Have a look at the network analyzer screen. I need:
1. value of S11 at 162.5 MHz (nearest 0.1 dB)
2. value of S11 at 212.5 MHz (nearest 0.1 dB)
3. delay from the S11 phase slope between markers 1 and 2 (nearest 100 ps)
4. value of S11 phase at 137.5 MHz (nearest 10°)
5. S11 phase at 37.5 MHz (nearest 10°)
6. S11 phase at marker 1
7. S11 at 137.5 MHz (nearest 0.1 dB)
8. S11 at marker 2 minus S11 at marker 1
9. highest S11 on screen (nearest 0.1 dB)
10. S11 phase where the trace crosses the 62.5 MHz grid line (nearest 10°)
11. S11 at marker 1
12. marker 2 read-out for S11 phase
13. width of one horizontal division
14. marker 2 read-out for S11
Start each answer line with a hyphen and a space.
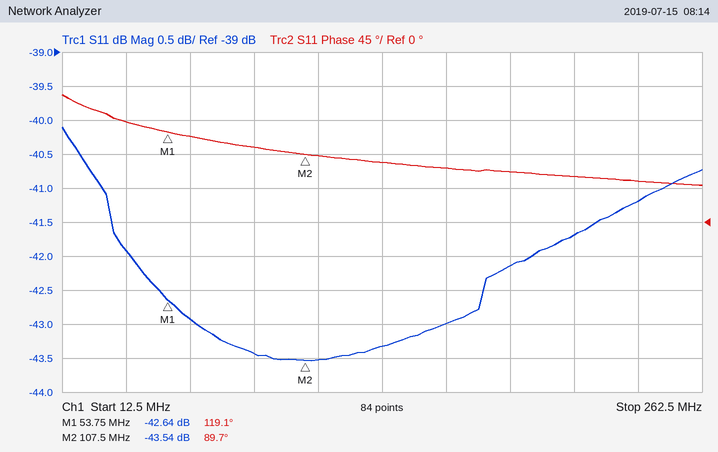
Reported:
- -43.0 dB
- -41.7 dB
- 1.5 ns
- 80°
- 130°
- 119.1°
- -43.3 dB
- -0.90 dB
- -40.1 dB
- 110°
- -42.64 dB
- 89.7°
- 25 MHz
- -43.54 dB
